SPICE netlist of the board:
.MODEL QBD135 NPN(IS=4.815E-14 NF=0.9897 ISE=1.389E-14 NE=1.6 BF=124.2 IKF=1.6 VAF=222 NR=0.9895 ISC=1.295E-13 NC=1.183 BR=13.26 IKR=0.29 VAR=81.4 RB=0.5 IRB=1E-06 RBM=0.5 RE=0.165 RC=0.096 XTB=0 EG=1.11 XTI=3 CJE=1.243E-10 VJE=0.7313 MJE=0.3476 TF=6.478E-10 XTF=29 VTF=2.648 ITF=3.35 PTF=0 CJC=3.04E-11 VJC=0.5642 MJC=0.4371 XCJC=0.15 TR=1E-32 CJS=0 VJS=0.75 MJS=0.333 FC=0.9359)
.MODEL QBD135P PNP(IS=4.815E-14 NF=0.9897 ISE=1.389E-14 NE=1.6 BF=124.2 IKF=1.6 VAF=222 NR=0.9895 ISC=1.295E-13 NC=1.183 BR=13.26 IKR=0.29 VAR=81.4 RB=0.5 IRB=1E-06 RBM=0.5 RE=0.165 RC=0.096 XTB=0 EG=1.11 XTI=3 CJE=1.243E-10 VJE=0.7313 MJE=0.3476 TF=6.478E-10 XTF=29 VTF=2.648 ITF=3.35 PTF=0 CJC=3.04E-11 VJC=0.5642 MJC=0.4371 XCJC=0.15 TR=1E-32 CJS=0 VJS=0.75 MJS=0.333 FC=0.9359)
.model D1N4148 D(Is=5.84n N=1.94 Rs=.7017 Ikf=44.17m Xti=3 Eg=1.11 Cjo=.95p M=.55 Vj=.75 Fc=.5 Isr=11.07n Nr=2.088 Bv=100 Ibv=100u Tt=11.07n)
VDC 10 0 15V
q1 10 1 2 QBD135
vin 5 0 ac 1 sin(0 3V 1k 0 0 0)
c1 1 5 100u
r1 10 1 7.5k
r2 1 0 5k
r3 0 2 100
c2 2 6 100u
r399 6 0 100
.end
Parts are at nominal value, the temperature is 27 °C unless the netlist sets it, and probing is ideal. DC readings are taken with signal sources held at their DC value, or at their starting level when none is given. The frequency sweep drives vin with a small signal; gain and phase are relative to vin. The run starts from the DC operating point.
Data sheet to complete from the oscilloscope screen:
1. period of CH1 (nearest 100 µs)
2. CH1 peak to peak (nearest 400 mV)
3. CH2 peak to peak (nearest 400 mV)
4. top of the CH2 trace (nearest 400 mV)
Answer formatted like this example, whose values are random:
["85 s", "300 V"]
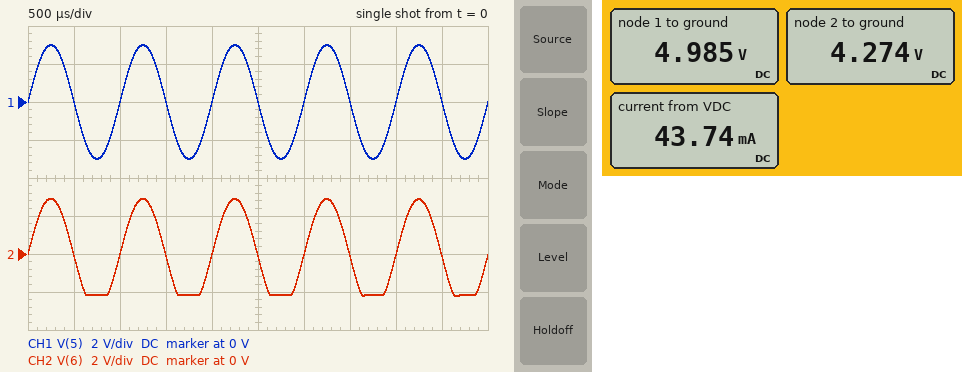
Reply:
["1.0 ms", "6.0 V", "5.2 V", "2.8 V"]
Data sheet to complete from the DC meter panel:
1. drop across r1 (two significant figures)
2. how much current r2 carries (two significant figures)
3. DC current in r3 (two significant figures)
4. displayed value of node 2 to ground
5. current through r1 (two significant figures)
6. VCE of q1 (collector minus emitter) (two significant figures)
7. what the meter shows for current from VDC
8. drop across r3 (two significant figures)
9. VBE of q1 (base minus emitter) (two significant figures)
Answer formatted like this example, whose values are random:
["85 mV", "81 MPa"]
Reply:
["10 V", "1.0 mA", "43 mA", "4.274 V", "1.3 mA", "11 V", "43.74 mA", "4.3 V", "710 mV"]
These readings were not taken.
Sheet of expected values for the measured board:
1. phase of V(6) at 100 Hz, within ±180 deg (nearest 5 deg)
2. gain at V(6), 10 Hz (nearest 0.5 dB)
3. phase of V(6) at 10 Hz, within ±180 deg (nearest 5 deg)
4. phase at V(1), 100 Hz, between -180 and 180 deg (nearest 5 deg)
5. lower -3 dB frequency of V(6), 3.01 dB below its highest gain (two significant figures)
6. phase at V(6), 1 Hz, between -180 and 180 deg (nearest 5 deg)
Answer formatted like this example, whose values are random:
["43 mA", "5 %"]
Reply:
["10 deg", "-5.5 dB", "60 deg", "0 deg", "16 Hz", "120 deg"]
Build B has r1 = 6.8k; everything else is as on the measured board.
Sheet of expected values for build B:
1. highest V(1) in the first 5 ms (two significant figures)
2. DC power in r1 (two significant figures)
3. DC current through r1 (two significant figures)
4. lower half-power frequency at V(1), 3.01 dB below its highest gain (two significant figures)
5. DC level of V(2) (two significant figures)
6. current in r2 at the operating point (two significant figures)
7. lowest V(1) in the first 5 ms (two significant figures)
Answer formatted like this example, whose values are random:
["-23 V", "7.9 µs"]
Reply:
["8.3 V", "14 mW", "1.4 mA", "690 mHz", "4.6 V", "1.1 mA", "2.3 V"]
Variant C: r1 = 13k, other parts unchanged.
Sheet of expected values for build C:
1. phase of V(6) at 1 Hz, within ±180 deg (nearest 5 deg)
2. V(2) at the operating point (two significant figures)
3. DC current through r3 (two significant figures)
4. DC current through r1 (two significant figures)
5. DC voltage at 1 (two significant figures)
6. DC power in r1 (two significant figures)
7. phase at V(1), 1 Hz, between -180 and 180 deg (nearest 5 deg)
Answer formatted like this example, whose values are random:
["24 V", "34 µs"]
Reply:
["115 deg", "2.7 V", "27 mA", "890 µA", "3.4 V", "10 mW", "30 deg"]
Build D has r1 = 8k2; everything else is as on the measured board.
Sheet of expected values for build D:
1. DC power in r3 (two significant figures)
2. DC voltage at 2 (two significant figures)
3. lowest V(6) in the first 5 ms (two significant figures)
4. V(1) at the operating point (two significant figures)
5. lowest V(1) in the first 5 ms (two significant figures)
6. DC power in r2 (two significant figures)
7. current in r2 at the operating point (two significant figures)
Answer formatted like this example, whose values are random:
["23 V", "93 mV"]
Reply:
["160 mW", "4.0 V", "-2.1 V", "4.7 V", "1.7 V", "4.4 mW", "940 µA"]
